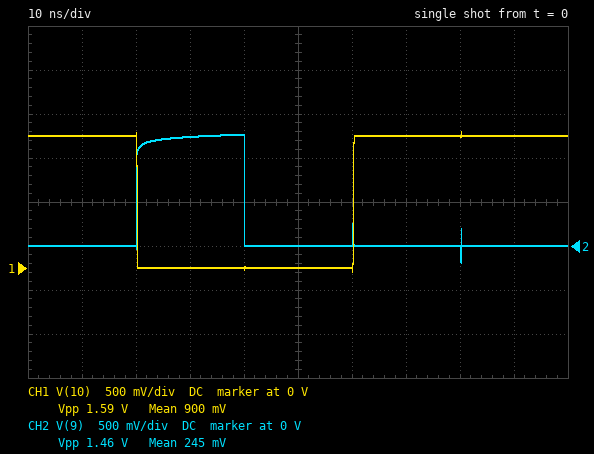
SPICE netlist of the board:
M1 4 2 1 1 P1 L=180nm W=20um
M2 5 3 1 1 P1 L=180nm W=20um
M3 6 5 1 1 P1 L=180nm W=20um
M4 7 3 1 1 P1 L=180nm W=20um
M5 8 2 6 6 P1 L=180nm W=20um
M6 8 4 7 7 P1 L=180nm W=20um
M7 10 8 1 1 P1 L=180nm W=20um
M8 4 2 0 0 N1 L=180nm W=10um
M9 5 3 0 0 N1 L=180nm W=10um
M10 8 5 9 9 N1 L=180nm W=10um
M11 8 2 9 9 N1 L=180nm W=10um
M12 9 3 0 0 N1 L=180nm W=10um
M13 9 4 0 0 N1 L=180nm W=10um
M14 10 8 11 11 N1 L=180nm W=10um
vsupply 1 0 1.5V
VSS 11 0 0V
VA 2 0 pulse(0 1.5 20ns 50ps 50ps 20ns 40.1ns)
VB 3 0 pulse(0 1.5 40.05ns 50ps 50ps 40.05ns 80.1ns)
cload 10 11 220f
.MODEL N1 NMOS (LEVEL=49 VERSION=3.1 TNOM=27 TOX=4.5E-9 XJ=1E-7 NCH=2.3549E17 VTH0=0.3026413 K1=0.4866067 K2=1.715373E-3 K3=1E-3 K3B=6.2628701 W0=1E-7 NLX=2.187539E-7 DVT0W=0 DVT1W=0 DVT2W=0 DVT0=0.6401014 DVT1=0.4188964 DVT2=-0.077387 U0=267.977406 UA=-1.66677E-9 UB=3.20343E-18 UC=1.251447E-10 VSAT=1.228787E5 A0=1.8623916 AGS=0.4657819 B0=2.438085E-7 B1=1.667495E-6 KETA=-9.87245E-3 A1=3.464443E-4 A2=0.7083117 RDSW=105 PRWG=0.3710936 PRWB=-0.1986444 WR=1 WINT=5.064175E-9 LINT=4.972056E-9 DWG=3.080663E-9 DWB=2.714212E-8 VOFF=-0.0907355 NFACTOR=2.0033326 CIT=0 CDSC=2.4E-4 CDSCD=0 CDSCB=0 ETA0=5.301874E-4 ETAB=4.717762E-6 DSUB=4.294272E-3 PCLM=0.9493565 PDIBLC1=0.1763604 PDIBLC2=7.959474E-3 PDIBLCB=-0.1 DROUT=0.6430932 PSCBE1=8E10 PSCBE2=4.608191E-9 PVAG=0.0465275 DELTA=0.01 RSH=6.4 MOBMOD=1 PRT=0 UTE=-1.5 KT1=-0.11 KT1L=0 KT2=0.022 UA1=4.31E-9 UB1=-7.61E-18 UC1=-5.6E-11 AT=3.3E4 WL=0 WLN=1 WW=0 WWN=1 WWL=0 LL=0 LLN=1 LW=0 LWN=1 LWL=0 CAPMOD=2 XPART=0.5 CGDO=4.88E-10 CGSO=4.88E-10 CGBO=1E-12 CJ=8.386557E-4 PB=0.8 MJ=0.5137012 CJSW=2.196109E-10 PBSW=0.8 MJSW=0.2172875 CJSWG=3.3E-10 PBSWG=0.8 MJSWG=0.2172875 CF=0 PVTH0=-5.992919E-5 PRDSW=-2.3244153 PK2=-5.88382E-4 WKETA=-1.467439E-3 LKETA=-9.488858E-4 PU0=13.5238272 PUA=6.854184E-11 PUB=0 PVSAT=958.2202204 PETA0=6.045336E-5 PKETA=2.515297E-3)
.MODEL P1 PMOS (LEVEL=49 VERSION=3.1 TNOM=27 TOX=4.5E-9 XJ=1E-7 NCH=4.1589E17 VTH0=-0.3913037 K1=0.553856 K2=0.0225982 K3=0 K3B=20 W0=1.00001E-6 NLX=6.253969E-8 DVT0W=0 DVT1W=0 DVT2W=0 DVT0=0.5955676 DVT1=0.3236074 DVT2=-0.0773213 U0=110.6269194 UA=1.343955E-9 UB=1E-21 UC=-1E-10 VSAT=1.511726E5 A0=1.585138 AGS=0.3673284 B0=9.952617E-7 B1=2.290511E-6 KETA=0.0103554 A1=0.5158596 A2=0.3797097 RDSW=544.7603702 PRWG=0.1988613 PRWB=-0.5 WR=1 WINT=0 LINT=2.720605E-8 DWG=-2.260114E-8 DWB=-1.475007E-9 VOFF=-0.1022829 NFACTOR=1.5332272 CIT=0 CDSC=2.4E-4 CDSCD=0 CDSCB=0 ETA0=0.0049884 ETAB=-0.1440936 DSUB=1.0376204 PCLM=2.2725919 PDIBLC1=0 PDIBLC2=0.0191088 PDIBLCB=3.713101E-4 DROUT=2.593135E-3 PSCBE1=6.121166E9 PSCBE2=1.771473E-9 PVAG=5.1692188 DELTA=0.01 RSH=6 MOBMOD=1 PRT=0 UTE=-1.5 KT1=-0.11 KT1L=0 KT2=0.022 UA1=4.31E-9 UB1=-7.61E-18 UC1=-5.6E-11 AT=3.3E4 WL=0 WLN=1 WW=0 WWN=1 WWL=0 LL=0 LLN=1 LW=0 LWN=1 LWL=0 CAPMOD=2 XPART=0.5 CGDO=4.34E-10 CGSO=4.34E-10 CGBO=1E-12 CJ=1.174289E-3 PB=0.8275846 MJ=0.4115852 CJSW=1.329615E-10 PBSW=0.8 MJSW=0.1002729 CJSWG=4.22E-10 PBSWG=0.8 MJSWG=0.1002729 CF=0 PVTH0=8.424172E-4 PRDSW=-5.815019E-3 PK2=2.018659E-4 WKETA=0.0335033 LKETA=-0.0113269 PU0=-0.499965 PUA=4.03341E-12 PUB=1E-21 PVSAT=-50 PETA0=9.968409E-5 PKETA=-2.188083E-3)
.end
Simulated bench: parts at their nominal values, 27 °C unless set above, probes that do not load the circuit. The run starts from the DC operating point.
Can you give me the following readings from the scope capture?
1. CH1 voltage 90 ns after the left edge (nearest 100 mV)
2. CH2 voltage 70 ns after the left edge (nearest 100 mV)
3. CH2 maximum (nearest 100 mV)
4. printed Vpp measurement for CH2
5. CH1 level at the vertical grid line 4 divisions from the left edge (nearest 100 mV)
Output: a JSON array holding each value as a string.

["1.5 V", "0 V", "1.3 V", "1.46 V", "0 V"]
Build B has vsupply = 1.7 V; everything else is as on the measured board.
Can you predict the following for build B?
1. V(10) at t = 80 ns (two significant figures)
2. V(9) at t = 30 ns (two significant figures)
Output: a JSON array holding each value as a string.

["1.7 V", "1.4 V"]
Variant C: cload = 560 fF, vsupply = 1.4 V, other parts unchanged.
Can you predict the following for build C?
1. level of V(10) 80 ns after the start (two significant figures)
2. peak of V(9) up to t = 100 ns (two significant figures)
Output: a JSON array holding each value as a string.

["1.4 V", "1.2 V"]
